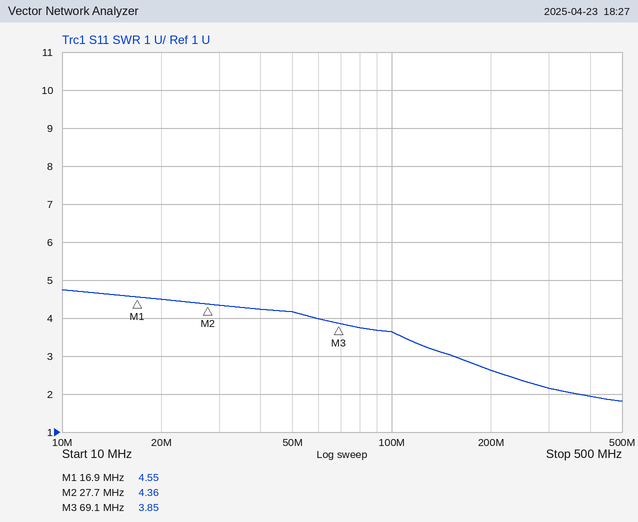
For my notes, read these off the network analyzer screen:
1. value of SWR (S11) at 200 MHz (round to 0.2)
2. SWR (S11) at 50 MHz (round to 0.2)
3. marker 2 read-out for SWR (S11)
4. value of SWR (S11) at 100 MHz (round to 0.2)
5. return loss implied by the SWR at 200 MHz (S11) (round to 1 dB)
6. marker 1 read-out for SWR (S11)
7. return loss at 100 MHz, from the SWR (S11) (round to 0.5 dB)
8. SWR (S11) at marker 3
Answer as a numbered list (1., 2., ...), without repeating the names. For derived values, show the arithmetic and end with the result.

1. 2.6
2. 4.2
3. 4.36
4. 3.6
5. −20 log10((2.6 − 1)/(2.6 + 1)) ≈ 7 dB
6. 4.55
7. −20 log10((3.6 − 1)/(3.6 + 1)) ≈ 5.0 dB
8. 3.85
